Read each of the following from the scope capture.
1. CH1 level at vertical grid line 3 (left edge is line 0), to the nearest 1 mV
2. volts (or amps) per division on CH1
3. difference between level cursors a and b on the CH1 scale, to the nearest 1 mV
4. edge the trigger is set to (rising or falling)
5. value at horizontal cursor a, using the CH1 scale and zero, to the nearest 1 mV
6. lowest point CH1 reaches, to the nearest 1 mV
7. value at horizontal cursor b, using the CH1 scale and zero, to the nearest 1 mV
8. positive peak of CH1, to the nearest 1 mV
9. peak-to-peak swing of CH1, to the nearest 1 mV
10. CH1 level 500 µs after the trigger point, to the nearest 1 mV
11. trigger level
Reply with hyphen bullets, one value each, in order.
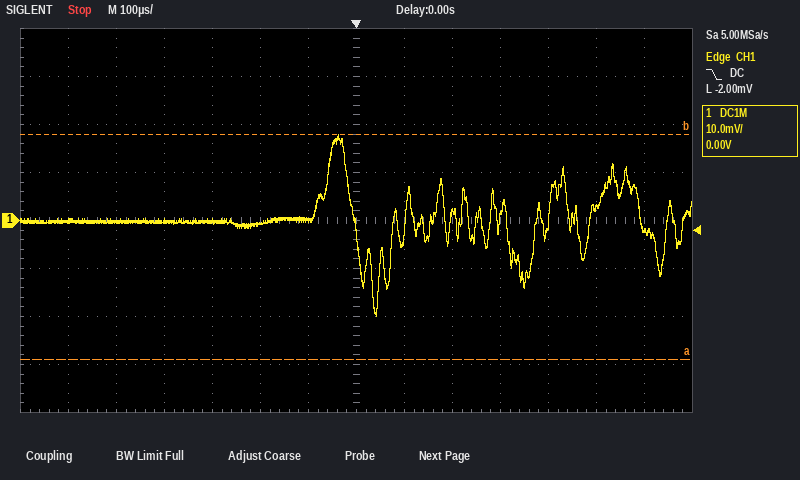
- 0 mV
- 10 mV
- 47 mV
- falling
- -29 mV
- -20 mV
- 18 mV
- 18 mV
- 38 mV
- 3 mV
- -2.00 mV
